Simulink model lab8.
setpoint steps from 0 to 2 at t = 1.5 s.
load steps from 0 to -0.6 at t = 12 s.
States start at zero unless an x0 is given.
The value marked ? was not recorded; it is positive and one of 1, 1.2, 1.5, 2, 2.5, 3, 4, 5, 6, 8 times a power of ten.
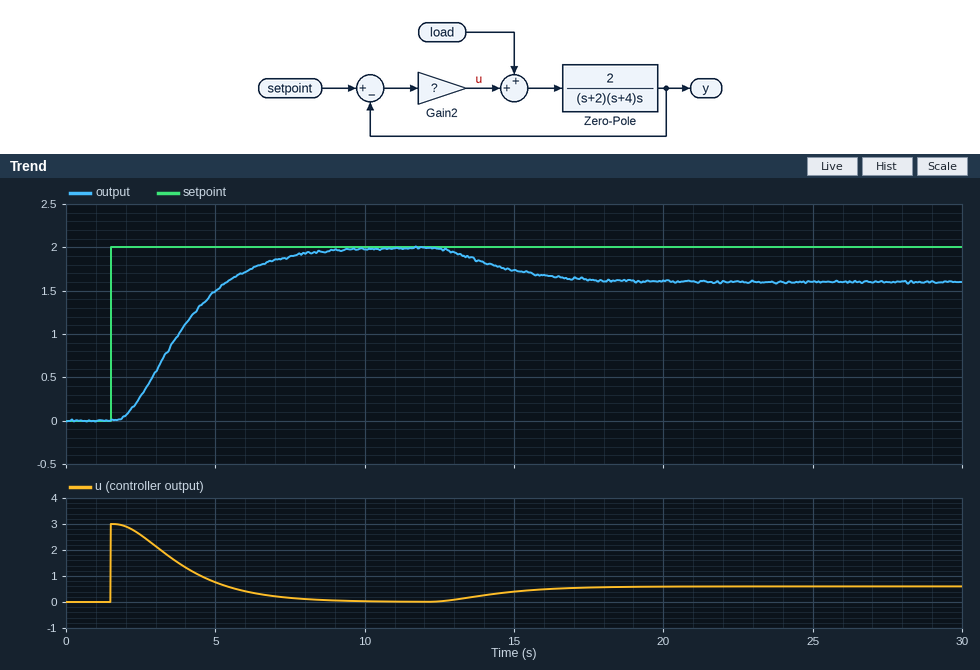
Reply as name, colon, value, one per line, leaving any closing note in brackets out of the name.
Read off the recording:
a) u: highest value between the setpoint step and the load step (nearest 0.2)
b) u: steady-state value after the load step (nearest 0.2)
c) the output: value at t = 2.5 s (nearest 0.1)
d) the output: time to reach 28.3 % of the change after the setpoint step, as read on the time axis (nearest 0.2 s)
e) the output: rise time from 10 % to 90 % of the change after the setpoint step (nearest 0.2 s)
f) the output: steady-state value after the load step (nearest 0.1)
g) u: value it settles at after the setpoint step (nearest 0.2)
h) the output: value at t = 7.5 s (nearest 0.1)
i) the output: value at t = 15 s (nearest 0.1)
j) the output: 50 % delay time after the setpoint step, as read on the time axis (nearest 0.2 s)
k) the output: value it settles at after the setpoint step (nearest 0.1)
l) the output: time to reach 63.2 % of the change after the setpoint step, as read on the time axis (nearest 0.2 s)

u: highest value between the setpoint step and the load step: 3.0
u: steady-state value after the load step: 0.6
the output: value at t = 2.5 s: 0.3
the output: time to reach 28.3 % of the change after the setpoint step, as read on the time axis: 3.0 s
the output: rise time from 10 % to 90 % of the change after the setpoint step: 4.2 s
the output: steady-state value after the load step: 1.6
u: value it settles at after the setpoint step: 0.0
the output: value at t = 7.5 s: 1.9
the output: value at t = 15 s: 1.7
the output: 50 % delay time after the setpoint step, as read on the time axis: 3.8 s
the output: value it settles at after the setpoint step: 2.0
the output: time to reach 63.2 % of the change after the setpoint step, as read on the time axis: 4.4 s
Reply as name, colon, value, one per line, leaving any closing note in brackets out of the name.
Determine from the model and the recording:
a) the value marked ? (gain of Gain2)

the value marked ?: 1.5
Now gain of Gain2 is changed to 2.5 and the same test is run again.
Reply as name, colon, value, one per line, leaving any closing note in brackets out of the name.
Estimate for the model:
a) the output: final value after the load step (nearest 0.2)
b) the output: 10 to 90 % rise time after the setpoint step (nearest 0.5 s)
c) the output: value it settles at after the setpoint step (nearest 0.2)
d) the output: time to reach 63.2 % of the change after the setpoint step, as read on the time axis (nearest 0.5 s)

the output: final value after the load step: 1.8
the output: 10 to 90 % rise time after the setpoint step: 2.0 s
the output: value it settles at after the setpoint step: 2.0
the output: time to reach 63.2 % of the change after the setpoint step, as read on the time axis: 3.5 s
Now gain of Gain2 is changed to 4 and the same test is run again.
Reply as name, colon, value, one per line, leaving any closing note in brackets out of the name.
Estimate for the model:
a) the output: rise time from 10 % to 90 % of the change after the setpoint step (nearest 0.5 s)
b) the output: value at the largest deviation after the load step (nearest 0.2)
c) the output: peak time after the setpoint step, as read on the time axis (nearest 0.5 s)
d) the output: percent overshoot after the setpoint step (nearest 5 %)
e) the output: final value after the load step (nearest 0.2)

the output: rise time from 10 % to 90 % of the change after the setpoint step: 1.5 s
the output: value at the largest deviation after the load step: 1.8
the output: peak time after the setpoint step, as read on the time axis: 4.5 s
the output: percent overshoot after the setpoint step: 15 %
the output: final value after the load step: 1.8
